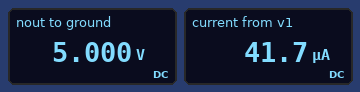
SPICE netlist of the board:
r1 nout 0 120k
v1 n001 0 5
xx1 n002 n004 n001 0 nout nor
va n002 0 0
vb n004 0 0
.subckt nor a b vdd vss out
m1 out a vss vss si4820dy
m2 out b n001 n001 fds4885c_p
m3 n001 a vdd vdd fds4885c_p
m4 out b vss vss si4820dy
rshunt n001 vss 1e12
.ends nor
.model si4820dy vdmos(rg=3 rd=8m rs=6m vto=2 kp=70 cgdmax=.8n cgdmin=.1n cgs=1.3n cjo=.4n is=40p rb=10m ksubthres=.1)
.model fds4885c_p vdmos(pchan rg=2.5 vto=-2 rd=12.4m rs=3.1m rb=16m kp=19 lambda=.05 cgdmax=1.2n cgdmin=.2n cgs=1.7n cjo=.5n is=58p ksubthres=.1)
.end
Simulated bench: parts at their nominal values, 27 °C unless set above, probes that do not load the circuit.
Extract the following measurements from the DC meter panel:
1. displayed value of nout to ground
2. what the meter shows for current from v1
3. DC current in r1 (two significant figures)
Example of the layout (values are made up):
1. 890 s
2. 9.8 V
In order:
1. 5.000 V
2. 41.7 µA
3. 42 µA
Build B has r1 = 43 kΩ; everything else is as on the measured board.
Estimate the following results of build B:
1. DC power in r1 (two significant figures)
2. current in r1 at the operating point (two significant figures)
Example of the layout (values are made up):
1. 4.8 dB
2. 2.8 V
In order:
1. 580 µW
2. 120 µA
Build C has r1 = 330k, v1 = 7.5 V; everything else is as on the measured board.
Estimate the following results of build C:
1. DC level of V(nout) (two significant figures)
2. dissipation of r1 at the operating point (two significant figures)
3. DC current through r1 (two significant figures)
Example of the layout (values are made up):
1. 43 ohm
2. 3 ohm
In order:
1. 7.5 V
2. 170 µW
3. 23 µA
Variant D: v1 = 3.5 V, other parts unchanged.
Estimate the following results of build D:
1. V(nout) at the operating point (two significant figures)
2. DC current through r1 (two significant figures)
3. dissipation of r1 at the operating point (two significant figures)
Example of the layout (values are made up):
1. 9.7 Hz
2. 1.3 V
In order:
1. 3.5 V
2. 29 µA
3. 100 µW
